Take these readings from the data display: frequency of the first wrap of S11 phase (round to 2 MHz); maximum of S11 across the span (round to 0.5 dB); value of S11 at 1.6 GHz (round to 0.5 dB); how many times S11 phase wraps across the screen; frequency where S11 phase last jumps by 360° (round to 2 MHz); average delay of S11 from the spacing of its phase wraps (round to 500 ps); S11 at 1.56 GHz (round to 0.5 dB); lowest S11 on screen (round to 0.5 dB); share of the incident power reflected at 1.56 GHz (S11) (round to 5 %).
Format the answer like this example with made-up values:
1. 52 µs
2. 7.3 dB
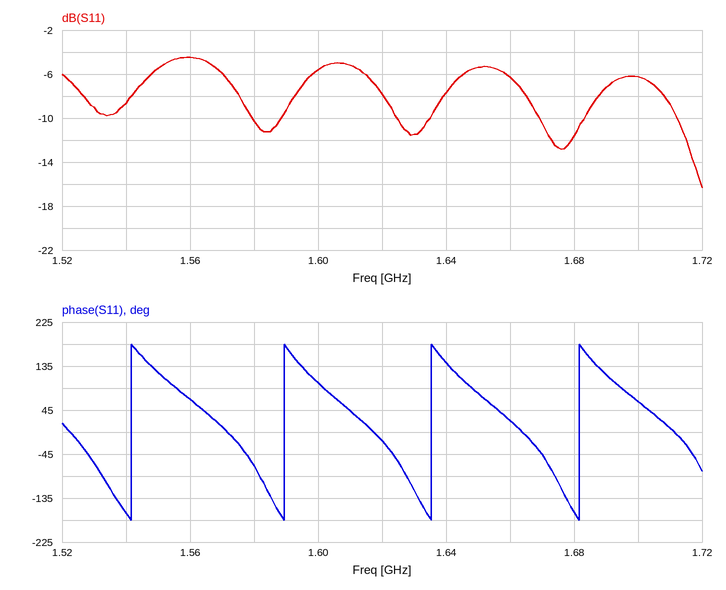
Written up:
1. 1.542 GHz
2. -4.5 dB
3. -5.5 dB
4. 4
5. 1.682 GHz
6. 21.5 ns
7. -4.5 dB
8. -16.5 dB
9. 35 %
